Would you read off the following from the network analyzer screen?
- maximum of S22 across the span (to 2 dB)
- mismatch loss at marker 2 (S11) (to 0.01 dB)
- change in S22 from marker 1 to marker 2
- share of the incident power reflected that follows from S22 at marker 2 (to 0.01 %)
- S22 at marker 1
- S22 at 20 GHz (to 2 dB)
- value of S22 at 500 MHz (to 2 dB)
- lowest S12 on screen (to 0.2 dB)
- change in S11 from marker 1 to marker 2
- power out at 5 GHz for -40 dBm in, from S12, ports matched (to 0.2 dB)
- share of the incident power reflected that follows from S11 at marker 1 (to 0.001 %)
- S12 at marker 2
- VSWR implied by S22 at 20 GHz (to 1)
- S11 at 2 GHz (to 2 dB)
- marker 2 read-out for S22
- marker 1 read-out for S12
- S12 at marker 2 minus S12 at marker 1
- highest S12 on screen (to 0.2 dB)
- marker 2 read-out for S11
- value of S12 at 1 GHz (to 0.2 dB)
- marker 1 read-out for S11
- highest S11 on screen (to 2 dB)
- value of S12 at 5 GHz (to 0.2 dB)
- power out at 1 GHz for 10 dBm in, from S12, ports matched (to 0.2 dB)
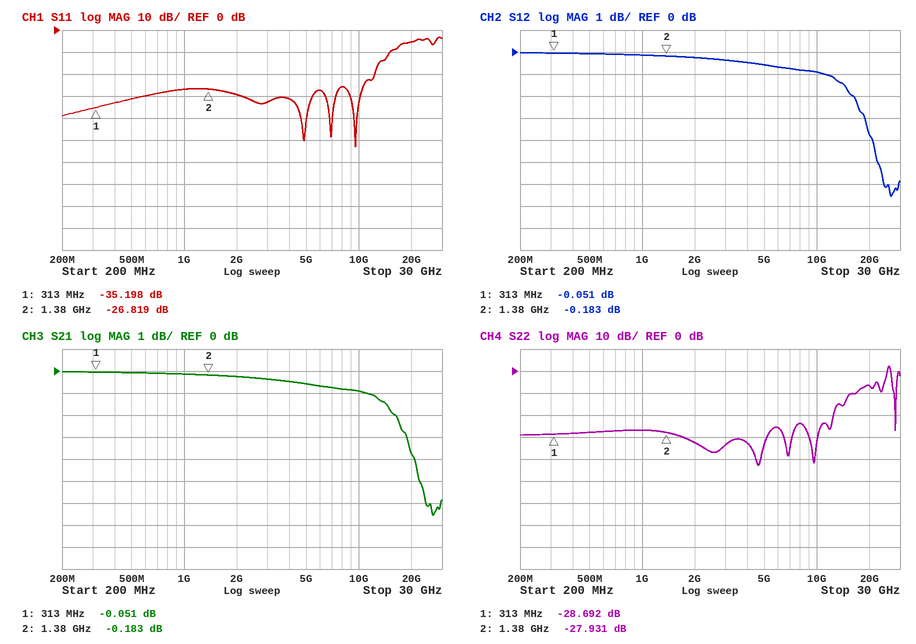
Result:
2 dB
0.01 dB
0.761 dB
0.16 %
-28.692 dB
-6 dB
-28 dB
-6.6 dB
8.379 dB
-40.6 dBm
0.030 %
-0.183 dB
3
-30 dB
-27.931 dB
-0.051 dB
-0.132 dB
0.0 dB
-26.819 dB
-0.2 dB
-35.198 dB
-4 dB
-0.6 dB
9.8 dBm
